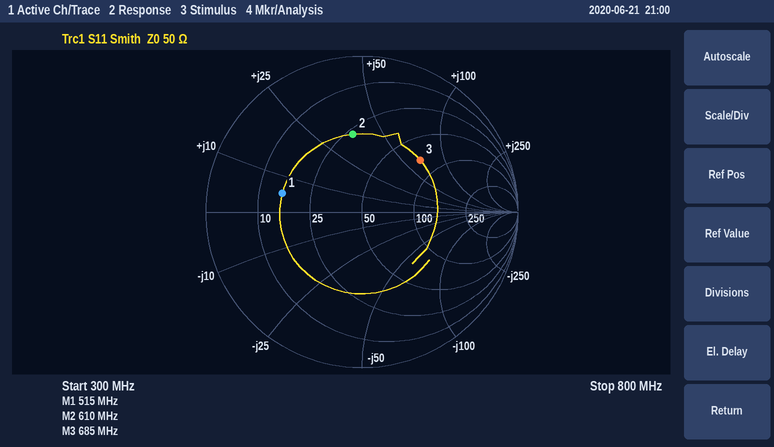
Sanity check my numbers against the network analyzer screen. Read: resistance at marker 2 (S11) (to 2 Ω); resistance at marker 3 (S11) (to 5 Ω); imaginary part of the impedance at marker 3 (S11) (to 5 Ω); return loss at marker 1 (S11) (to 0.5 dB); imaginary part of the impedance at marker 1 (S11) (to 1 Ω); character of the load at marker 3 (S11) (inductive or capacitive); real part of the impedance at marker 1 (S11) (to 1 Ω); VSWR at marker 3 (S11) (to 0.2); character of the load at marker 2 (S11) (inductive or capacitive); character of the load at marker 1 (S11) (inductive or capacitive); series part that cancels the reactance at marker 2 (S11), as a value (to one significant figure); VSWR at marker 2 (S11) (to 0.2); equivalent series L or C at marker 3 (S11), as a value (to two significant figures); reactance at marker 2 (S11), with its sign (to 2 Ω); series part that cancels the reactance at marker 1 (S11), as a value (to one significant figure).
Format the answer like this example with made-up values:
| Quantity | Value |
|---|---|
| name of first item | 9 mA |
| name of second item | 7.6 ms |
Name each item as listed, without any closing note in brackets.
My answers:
| Quantity | Value |
|---|---|
| resistance at marker 2 (S11) | 28 Ω |
| resistance at marker 3 (S11) | 75 Ω |
| imaginary part of the impedance at marker 3 (S11) | +65 Ω |
| return loss at marker 1 (S11) | 5.5 dB |
| imaginary part of the impedance at marker 1 (S11) | +5 Ω |
| character of the load at marker 3 (S11) | inductive |
| real part of the impedance at marker 1 (S11) | 16 Ω |
| VSWR at marker 3 (S11) | 3.0 |
| character of the load at marker 2 (S11) | inductive |
| character of the load at marker 1 (S11) | inductive |
| series part that cancels the reactance at marker 2 (S11), as a value | 7 pF |
| VSWR at marker 2 (S11) | 3.0 |
| equivalent series L or C at marker 3 (S11), as a value | 15 nH |
| reactance at marker 2 (S11), with its sign | +36 Ω |
| series part that cancels the reactance at marker 1 (S11), as a value | 60 pF |
